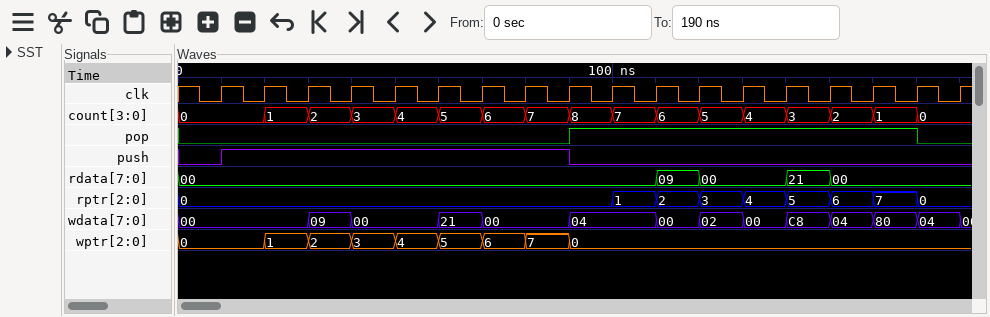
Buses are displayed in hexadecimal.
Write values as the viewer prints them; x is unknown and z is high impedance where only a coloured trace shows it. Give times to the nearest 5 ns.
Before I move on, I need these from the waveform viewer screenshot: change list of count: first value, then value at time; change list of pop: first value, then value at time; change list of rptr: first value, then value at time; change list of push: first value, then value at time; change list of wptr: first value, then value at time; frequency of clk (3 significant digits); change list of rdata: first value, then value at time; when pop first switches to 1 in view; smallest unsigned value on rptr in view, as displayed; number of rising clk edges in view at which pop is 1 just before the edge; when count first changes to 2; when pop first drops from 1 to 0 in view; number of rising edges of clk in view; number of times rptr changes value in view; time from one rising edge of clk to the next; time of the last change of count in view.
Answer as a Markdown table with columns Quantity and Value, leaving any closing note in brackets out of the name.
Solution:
| Quantity | Value |
|---|---|
| change list of count: first value, then value at time | 0, 1 at 20 ns, 2 at 30 ns, 3 at 40 ns, 4 at 50 ns, 5 at 60 ns, 6 at 70 ns, 7 at 80 ns, 8 at 90 ns, 7 at 100 ns, 6 at 110 ns, 5 at 120 ns, 4 at 130 ns, 3 at 140 ns, 2 at 150 ns, 1 at 160 ns, 0 at 170 ns |
| change list of pop: first value, then value at time | 0, 1 at 90 ns, 0 at 170 ns |
| change list of rptr: first value, then value at time | 0, 1 at 100 ns, 2 at 110 ns, 3 at 120 ns, 4 at 130 ns, 5 at 140 ns, 6 at 150 ns, 7 at 160 ns, 0 at 170 ns |
| change list of push: first value, then value at time | 0, 1 at 10 ns, 0 at 90 ns |
| change list of wptr: first value, then value at time | 0, 1 at 20 ns, 2 at 30 ns, 3 at 40 ns, 4 at 50 ns, 5 at 60 ns, 6 at 70 ns, 7 at 80 ns, 0 at 90 ns |
| frequency of clk | 100 MHz |
| change list of rdata: first value, then value at time | 00, 09 at 110 ns, 00 at 120 ns, 21 at 140 ns, 00 at 150 ns |
| when pop first switches to 1 in view | 90 ns |
| smallest unsigned value on rptr in view, as displayed | 0 |
| number of rising clk edges in view at which pop is 1 just before the edge | 8 |
| when count first changes to 2 | 30 ns |
| when pop first drops from 1 to 0 in view | 170 ns |
| number of rising edges of clk in view | 18 |
| number of times rptr changes value in view | 8 |
| time from one rising edge of clk to the next | 10 ns |
| time of the last change of count in view | 170 ns |
